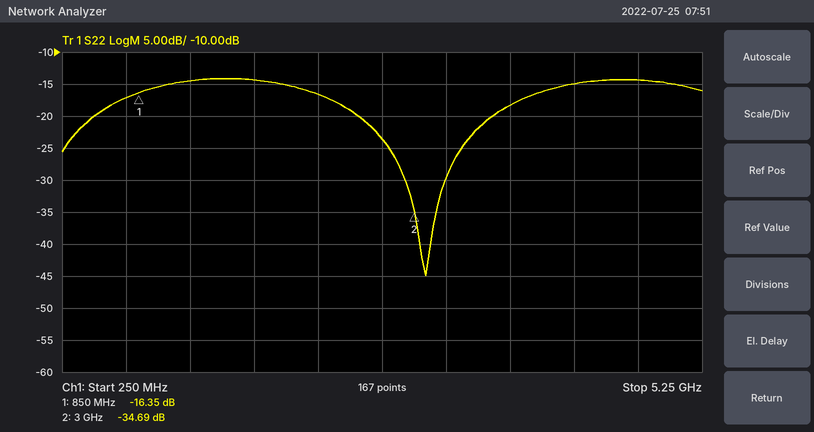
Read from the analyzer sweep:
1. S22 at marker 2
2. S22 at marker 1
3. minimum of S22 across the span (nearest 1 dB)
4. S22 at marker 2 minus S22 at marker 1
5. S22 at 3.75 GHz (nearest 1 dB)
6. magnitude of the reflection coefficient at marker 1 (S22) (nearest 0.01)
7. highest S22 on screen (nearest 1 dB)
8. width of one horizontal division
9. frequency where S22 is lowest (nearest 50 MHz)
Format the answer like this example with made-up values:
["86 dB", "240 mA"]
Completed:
["-34.69 dB", "-16.35 dB", "-45 dB", "-18.34 dB", "-18 dB", "0.15", "-14 dB", "500 MHz", "3.10 GHz"]
